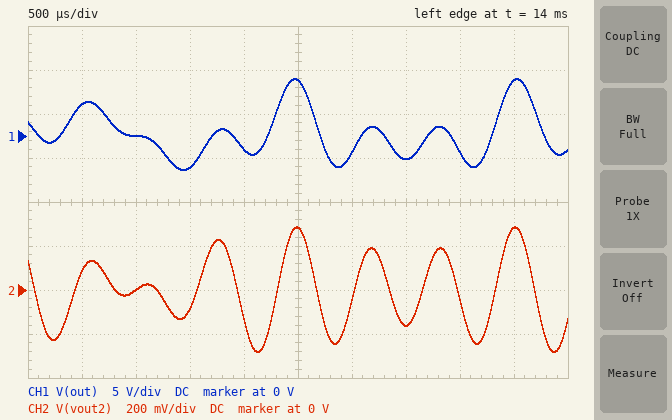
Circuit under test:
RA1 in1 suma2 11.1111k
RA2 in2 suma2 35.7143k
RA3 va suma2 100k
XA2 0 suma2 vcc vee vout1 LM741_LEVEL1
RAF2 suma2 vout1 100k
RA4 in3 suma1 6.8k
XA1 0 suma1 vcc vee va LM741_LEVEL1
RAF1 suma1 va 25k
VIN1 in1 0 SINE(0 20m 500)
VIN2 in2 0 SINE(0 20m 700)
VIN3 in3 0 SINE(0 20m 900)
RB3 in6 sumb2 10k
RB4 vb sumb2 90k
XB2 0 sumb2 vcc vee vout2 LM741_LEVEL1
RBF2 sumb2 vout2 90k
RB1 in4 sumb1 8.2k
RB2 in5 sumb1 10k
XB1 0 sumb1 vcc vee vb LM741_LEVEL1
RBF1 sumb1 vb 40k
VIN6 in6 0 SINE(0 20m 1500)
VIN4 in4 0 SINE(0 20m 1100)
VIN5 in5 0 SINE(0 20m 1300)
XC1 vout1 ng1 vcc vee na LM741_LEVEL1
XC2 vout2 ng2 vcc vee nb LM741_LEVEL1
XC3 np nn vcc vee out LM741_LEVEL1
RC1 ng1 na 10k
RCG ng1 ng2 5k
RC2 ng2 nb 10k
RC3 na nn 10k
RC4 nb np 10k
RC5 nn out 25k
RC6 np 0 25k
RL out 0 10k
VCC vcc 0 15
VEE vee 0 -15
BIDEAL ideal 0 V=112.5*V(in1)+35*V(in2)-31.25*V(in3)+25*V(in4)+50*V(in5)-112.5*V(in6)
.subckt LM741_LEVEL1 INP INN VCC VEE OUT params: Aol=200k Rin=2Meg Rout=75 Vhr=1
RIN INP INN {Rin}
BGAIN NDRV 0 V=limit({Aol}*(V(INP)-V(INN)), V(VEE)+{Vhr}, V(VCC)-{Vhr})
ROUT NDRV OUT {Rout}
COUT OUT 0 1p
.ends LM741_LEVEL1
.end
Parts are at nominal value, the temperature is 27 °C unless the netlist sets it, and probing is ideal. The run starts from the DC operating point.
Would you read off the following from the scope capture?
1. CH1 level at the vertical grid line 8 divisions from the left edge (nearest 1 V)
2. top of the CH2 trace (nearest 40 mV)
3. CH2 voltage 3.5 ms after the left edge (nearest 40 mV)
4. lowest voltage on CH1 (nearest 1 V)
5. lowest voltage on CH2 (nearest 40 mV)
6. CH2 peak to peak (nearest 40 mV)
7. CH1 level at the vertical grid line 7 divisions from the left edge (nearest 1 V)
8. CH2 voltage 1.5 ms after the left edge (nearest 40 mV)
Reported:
-2 V
280 mV
-160 mV
-4 V
-280 mV
560 mV
-3 V
-80 mV
